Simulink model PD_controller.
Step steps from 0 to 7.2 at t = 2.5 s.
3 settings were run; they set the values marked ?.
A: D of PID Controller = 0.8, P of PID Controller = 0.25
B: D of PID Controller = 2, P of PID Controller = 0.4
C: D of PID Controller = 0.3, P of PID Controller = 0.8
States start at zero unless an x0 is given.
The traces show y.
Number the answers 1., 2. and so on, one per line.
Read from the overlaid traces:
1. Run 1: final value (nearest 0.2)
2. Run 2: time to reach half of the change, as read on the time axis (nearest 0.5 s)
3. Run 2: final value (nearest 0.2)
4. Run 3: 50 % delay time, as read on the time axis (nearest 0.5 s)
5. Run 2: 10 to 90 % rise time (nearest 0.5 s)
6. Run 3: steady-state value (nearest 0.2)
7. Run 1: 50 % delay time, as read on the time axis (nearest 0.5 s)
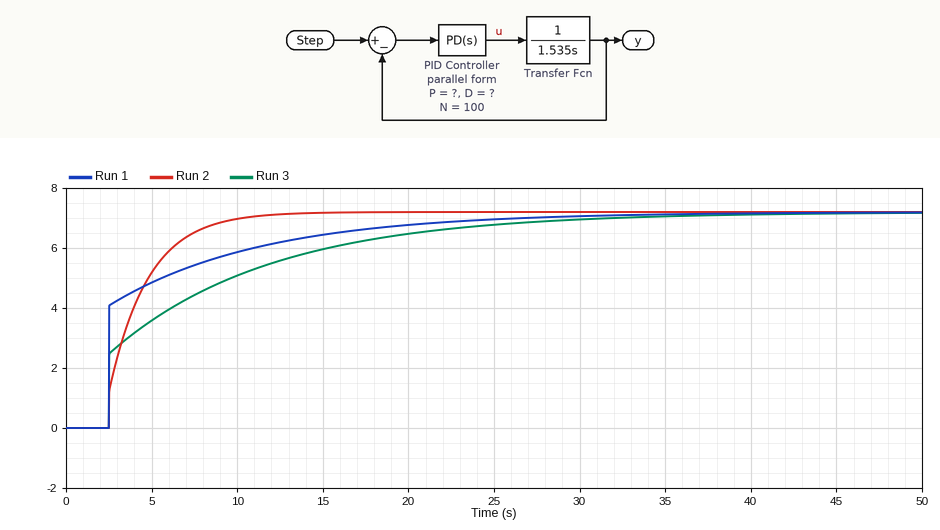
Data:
1. 7.2
2. 3.5 s
3. 7.2
4. 5.0 s
5. 5.0 s
6. 7.2
7. 2.5 s
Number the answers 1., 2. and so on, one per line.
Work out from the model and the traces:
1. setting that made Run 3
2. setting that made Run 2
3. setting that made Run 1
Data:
1. A
2. C
3. B
